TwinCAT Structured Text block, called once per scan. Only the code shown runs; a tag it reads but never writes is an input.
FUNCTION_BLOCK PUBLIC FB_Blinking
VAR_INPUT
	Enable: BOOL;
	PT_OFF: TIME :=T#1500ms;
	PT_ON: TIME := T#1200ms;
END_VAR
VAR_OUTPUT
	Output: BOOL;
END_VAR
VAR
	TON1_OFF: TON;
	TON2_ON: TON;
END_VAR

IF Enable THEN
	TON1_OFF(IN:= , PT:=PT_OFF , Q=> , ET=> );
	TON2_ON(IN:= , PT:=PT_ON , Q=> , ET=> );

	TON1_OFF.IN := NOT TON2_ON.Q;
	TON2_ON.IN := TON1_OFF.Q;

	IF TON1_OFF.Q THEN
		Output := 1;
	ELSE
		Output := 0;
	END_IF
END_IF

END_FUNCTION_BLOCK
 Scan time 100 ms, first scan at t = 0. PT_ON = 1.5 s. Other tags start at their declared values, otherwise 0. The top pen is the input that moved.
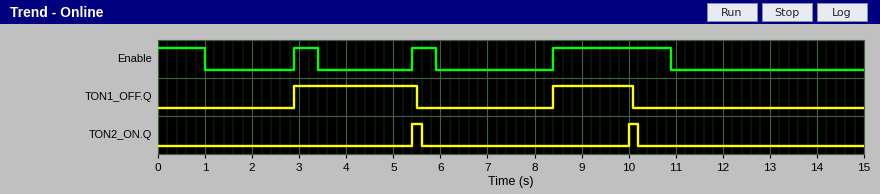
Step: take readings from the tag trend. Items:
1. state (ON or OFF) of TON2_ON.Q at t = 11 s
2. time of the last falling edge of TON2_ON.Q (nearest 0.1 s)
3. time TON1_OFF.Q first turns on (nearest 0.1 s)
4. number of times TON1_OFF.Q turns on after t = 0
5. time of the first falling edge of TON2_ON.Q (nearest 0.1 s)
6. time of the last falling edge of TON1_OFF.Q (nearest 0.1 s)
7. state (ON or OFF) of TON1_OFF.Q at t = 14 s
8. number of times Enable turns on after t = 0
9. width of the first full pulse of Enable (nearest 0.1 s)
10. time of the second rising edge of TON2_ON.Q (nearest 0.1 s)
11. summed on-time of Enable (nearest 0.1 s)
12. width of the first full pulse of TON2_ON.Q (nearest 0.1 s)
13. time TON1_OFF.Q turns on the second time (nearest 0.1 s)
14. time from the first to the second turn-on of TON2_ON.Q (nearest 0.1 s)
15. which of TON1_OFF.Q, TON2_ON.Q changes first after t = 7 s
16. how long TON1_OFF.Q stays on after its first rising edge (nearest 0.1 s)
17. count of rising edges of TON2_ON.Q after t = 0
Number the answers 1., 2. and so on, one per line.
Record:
1. OFF
2. 10.2 s
3. 2.9 s
4. 2
5. 5.6 s
6. 10.1 s
7. OFF
8. 3
9. 0.5 s
10. 10.0 s
11. 4.5 s
12. 0.2 s
13. 8.4 s
14. 4.6 s
15. TON1_OFF.Q
16. 2.6 s
17. 2
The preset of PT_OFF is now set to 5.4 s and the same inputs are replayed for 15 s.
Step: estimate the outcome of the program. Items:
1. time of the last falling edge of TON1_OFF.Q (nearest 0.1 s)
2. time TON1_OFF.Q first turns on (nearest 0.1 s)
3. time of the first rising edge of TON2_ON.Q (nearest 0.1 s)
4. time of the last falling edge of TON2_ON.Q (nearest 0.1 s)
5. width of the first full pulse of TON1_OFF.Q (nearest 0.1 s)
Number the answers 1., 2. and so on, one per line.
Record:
1. 8.5 s
2. 5.5 s
3. 8.4 s
4. 8.6 s
5. 3.0 s
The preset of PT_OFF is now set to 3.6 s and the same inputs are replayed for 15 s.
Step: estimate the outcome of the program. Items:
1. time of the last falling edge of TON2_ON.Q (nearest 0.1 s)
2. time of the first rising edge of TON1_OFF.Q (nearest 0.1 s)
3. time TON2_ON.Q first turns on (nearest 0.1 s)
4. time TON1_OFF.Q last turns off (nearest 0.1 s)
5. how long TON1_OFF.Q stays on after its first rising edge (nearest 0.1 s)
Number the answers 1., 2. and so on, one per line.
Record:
1. 8.6 s
2. 5.4 s
3. 8.4 s
4. 8.5 s
5. 3.1 s
